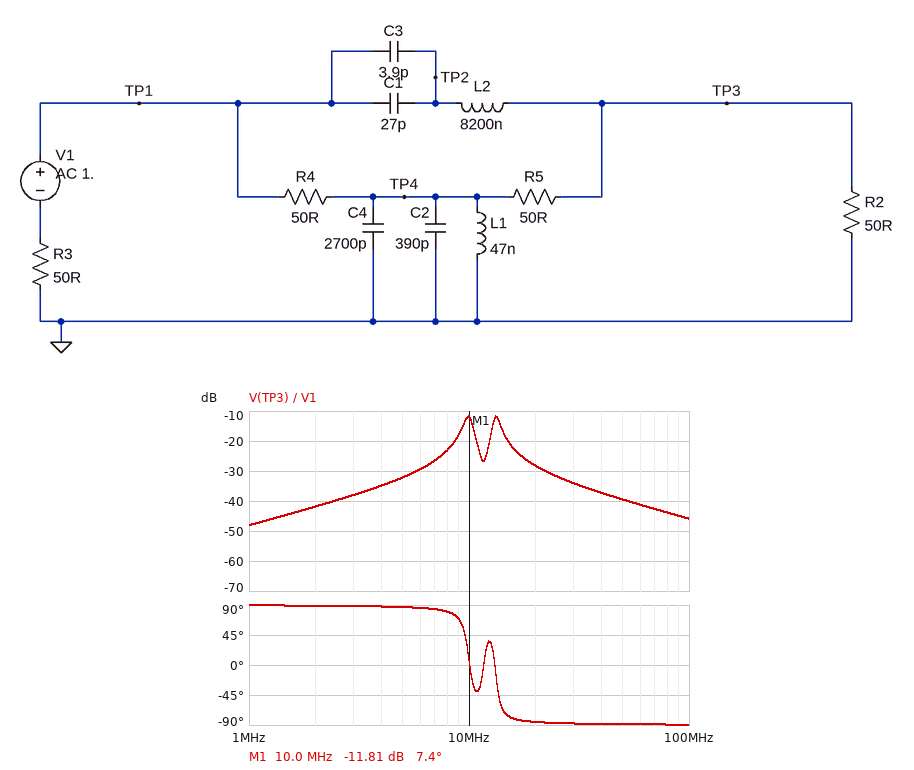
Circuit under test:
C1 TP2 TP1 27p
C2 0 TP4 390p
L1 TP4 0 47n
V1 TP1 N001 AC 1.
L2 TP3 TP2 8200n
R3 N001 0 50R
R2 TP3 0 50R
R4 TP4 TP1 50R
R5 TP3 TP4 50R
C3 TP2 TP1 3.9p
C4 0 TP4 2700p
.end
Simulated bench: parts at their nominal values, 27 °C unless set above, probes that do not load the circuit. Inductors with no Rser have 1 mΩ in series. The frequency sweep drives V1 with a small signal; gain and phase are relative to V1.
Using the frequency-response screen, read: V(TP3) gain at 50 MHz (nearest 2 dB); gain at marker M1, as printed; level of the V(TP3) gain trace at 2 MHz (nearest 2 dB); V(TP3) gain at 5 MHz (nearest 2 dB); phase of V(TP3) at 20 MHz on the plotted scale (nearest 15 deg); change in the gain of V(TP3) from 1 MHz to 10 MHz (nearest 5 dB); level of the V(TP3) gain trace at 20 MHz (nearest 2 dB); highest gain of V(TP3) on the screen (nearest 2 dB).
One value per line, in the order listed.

-40 dB
-11.81 dB
-42 dB
-32 dB
-90 deg
35 dB
-28 dB
-12 dB
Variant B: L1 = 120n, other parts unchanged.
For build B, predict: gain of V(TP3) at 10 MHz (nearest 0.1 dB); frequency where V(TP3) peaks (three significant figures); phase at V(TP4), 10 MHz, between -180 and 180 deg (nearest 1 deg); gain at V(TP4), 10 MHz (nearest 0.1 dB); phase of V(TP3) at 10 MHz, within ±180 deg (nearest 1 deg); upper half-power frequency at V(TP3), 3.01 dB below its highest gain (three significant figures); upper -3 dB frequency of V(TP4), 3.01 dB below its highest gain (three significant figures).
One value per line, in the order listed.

-10.9 dB
10.1 MHz
-72 deg
-16.2 dB
-15 deg
10.7 MHz
8.80 MHz
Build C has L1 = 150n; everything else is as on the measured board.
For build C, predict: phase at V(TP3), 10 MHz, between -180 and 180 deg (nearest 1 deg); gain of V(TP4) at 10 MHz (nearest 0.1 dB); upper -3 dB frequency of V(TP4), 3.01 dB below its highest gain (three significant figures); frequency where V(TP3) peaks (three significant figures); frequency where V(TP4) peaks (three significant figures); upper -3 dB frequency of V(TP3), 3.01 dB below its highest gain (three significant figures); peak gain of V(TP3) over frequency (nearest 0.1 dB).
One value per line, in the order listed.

-12 deg
-19.1 dB
7.93 MHz
10.1 MHz
7.39 MHz
10.7 MHz
-11.3 dB
